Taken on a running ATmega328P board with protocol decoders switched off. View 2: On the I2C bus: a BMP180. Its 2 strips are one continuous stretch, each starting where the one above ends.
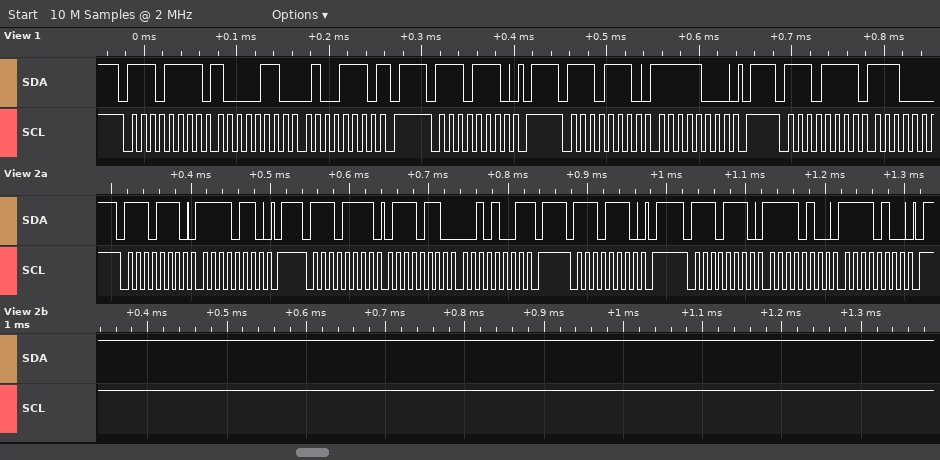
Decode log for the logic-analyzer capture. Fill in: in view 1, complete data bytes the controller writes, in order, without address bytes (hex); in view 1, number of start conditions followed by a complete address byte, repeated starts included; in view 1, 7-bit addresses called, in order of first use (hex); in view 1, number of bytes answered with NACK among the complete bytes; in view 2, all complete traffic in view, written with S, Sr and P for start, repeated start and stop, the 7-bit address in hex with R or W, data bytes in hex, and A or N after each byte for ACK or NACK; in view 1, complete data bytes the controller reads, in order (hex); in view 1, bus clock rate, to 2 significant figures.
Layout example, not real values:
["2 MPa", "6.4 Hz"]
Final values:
["F8", "4", "0x77", "1", "S 77W A F6 A P S 77R A 76 A 29 N P S 77W A P S 77W A F4 A F4 A P", "86 4E", "100 kHz"]
